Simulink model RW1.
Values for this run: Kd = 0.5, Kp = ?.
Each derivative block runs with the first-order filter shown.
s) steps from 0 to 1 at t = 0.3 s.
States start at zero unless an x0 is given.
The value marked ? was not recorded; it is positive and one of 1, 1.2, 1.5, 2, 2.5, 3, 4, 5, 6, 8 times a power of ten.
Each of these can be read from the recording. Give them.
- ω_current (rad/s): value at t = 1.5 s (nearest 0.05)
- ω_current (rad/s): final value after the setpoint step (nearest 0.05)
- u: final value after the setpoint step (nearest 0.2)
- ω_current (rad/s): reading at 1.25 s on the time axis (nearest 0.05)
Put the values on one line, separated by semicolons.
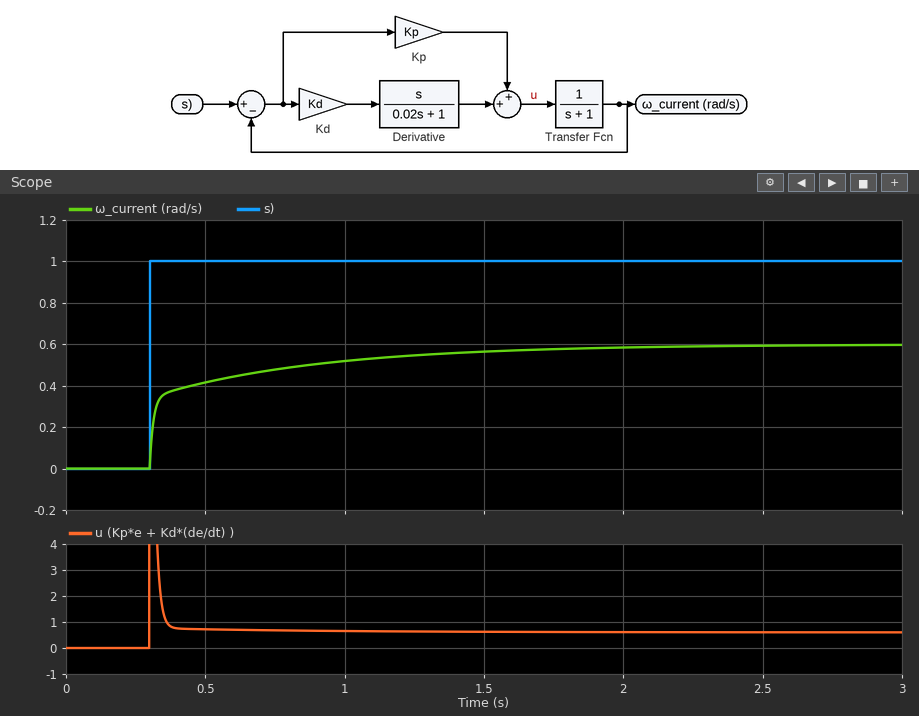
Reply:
0.55; 0.60; 0.6; 0.55
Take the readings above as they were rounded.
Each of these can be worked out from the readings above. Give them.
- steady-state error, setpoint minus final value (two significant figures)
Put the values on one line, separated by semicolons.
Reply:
0.40
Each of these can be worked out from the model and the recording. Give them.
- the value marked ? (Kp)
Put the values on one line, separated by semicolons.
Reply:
1.5
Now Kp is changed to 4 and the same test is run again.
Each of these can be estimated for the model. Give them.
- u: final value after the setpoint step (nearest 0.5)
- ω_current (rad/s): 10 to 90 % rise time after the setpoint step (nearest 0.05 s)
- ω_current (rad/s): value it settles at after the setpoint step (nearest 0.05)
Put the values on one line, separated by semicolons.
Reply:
1.0; 0.50 s; 0.80
